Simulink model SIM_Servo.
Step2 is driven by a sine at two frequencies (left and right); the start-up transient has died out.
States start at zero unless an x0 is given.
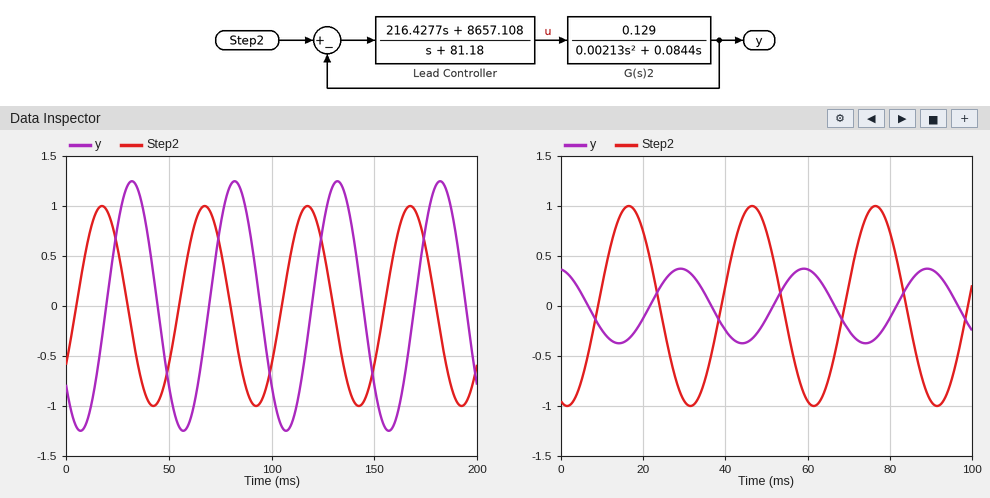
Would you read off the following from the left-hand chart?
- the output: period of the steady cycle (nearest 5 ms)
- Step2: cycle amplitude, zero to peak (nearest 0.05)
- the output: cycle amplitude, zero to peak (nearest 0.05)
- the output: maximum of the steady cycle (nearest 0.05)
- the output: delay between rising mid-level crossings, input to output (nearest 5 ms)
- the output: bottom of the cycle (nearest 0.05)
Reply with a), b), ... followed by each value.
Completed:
a) 50 ms
b) 1.00
c) 1.25
d) 1.25
e) 15 ms
f) -1.25
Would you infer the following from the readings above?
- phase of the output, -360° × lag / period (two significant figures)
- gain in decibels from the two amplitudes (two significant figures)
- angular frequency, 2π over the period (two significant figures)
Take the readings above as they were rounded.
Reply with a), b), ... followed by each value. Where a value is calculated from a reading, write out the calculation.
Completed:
a) -360 × 15 / 50 = -110°
b) 20 log10(1.25 / 1) = 1.9 dB
c) 2π / 50 = 0.13 rad/ms
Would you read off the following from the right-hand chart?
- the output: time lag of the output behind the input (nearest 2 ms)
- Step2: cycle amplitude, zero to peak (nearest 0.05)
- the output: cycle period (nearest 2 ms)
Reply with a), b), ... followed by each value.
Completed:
a) 12 ms
b) 1.00
c) 30 ms
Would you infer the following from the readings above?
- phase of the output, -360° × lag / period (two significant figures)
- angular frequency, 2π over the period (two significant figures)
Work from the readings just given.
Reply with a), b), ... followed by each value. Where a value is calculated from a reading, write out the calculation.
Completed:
a) -360 × 12 / 30 = -140°
b) 2π / 30 = 0.21 rad/ms
